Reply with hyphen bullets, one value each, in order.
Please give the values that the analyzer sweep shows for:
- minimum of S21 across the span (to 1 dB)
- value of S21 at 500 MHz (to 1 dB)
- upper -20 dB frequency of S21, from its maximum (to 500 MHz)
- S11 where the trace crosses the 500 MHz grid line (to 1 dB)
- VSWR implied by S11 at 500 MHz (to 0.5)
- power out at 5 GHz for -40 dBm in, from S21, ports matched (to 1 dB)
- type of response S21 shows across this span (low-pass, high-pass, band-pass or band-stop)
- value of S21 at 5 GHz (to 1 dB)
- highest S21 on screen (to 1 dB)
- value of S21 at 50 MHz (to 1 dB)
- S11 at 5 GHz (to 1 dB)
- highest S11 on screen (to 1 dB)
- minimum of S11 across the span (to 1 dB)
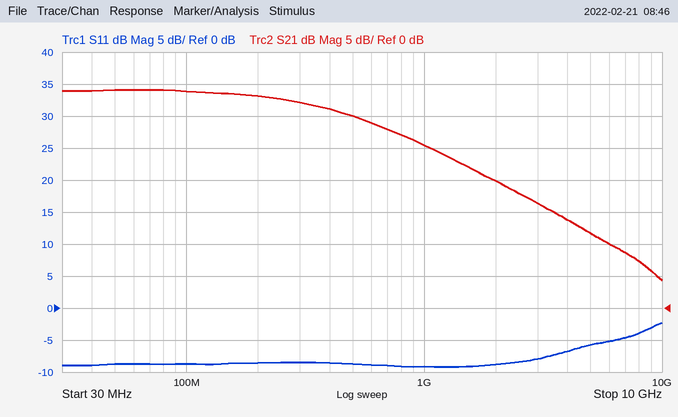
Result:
- 4 dB
- 30 dB
- 4.0 GHz
- -9 dB
- 2.0
- -28 dBm
- low-pass
- 12 dB
- 34 dB
- 34 dB
- -6 dB
- -2 dB
- -9 dB
